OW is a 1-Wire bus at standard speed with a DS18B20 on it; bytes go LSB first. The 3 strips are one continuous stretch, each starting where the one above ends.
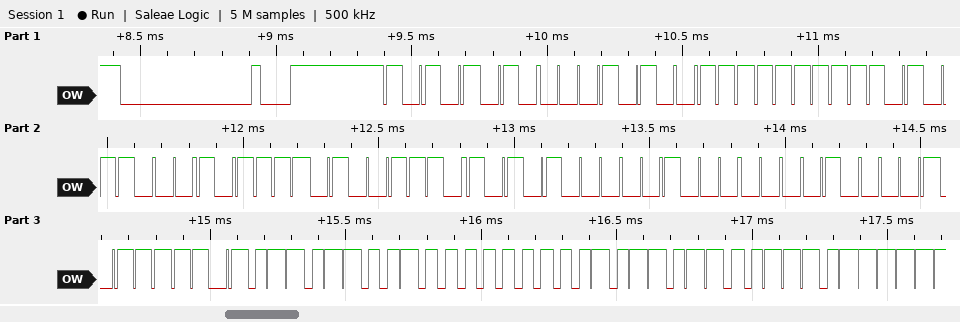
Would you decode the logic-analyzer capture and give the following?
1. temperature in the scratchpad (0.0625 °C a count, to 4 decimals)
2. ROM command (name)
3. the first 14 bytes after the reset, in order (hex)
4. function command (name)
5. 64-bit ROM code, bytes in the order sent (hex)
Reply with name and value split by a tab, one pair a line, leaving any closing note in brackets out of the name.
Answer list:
temperature in the scratchpad	19.3750 °C
ROM command	Match ROM
the first 14 bytes after the reset, in order	55 28 FF 6B F4 72 15 04 84 BE 36 01 B4 B9
function command	Read Scratchpad
64-bit ROM code, bytes in the order sent	28 FF 6B F4 72 15 04 84
